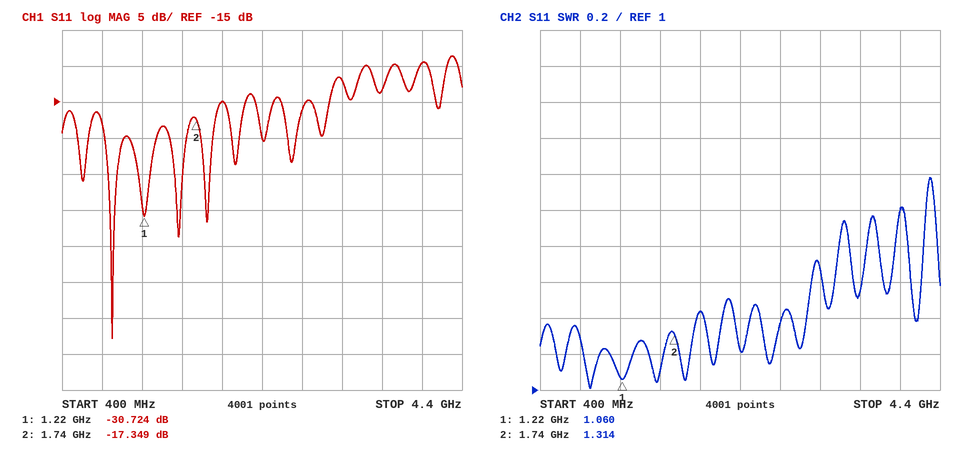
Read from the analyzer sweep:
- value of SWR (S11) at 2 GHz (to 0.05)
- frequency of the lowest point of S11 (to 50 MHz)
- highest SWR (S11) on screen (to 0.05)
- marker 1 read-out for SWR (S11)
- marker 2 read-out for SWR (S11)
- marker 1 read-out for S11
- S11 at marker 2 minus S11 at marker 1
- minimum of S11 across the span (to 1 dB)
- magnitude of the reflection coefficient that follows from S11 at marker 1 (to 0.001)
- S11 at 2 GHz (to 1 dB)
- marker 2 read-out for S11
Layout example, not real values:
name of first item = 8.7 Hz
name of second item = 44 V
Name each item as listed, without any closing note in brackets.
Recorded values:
value of SWR (S11) at 2 GHz = 1.45
frequency of the lowest point of S11 = 900 MHz
highest SWR (S11) on screen = 2.20
marker 1 read-out for SWR = 1.060
marker 2 read-out for SWR = 1.314
marker 1 read-out for S11 = -30.724 dB
S11 at marker 2 minus S11 at marker 1 = 13.375 dB
minimum of S11 across the span = -48 dB
magnitude of the reflection coefficient that follows from S11 at marker 1 = 0.029
S11 at 2 GHz = -15 dB
marker 2 read-out for S11 = -17.349 dB
